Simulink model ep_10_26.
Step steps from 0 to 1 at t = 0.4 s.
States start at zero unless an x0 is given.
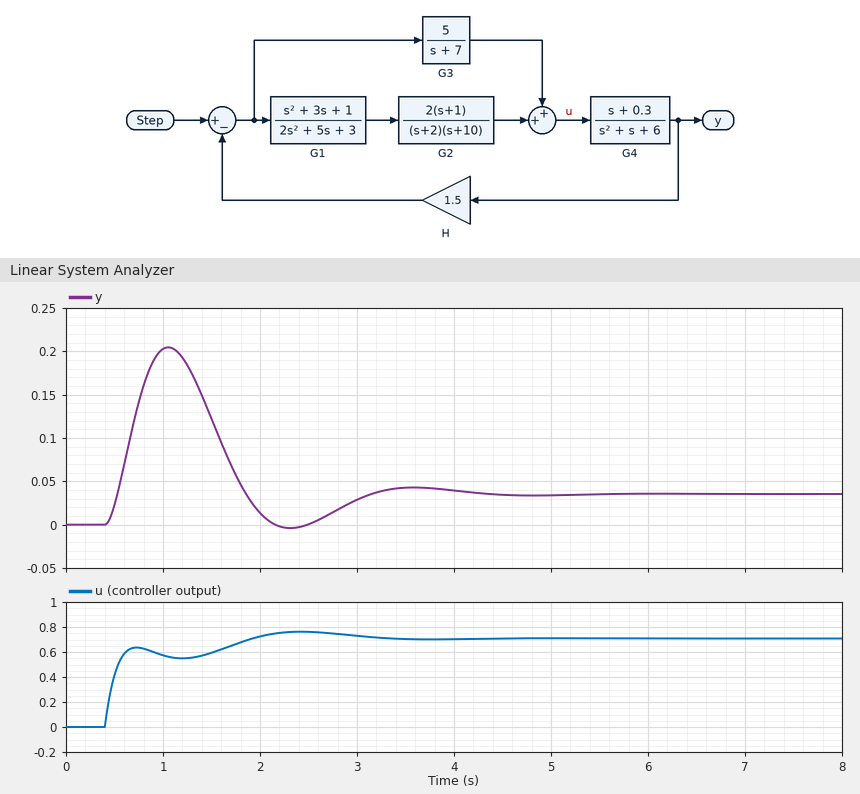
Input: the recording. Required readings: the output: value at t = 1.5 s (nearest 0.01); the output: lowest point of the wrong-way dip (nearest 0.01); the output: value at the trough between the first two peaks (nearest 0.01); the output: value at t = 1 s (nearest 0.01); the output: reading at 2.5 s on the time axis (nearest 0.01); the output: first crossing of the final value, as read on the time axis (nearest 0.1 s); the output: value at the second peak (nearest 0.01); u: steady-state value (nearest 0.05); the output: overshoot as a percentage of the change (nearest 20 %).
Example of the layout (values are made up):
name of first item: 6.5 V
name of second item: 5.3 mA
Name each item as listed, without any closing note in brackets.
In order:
the output: value at t = 1.5 s: 0.12
the output: lowest point of the wrong-way dip: 0.00
the output: value at the trough between the first two peaks: 0.00
the output: value at t = 1 s: 0.20
the output: reading at 2.5 s on the time axis: 0.00
the output: first crossing of the final value, as read on the time axis: 0.5 s
the output: value at the second peak: 0.04
u: steady-state value: 0.70
the output: overshoot as a percentage of the change: 480 %
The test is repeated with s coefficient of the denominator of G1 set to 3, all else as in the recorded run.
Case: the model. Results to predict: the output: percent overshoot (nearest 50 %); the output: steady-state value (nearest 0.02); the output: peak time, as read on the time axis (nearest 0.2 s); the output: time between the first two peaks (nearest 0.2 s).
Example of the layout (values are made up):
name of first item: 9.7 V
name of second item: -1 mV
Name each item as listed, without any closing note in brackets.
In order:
the output: percent overshoot: 500 %
the output: steady-state value: 0.04
the output: peak time, as read on the time axis: 1.0 s
the output: time between the first two peaks: 2.6 s
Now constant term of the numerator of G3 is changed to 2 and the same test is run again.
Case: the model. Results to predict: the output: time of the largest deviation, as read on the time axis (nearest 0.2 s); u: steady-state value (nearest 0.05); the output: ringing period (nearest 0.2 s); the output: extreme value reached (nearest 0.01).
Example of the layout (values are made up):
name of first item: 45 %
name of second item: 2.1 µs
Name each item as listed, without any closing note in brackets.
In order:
the output: time of the largest deviation, as read on the time axis: 1.0 s
u: steady-state value: 0.30
the output: ringing period: 2.6 s
the output: extreme value reached: 0.11
